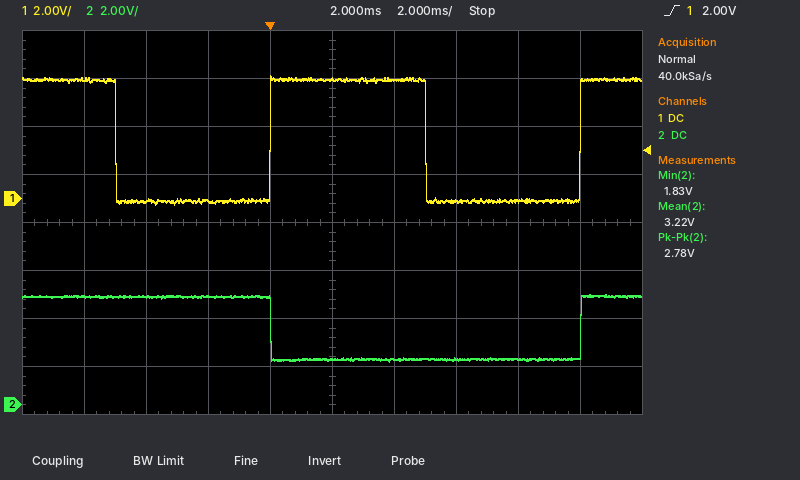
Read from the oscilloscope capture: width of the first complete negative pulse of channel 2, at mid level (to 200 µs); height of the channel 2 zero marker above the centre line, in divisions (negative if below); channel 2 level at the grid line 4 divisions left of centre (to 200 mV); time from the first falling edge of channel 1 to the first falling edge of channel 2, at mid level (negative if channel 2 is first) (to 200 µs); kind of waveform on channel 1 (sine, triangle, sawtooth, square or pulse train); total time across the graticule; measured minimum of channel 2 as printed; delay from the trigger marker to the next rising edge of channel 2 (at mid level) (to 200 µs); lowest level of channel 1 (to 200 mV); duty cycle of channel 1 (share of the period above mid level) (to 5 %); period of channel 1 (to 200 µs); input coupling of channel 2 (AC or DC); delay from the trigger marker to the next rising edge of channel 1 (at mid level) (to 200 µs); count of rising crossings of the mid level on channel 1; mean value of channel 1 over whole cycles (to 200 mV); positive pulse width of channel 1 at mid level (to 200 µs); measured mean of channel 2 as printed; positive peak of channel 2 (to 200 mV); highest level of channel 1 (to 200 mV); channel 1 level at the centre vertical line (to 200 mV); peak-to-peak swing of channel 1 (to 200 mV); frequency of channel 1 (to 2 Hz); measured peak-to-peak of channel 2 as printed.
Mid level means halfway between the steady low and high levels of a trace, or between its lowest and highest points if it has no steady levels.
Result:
10.0 ms
-3.8 div
4.6 V
+5.0 ms
square
20 ms
1.83 V
10.0 ms
-200 mV
50 %
10.0 ms
DC
10.0 ms
2
2.4 V
5.0 ms
3.22 V
4.6 V
5.2 V
5.0 V
5.4 V
100 Hz
2.78 V
